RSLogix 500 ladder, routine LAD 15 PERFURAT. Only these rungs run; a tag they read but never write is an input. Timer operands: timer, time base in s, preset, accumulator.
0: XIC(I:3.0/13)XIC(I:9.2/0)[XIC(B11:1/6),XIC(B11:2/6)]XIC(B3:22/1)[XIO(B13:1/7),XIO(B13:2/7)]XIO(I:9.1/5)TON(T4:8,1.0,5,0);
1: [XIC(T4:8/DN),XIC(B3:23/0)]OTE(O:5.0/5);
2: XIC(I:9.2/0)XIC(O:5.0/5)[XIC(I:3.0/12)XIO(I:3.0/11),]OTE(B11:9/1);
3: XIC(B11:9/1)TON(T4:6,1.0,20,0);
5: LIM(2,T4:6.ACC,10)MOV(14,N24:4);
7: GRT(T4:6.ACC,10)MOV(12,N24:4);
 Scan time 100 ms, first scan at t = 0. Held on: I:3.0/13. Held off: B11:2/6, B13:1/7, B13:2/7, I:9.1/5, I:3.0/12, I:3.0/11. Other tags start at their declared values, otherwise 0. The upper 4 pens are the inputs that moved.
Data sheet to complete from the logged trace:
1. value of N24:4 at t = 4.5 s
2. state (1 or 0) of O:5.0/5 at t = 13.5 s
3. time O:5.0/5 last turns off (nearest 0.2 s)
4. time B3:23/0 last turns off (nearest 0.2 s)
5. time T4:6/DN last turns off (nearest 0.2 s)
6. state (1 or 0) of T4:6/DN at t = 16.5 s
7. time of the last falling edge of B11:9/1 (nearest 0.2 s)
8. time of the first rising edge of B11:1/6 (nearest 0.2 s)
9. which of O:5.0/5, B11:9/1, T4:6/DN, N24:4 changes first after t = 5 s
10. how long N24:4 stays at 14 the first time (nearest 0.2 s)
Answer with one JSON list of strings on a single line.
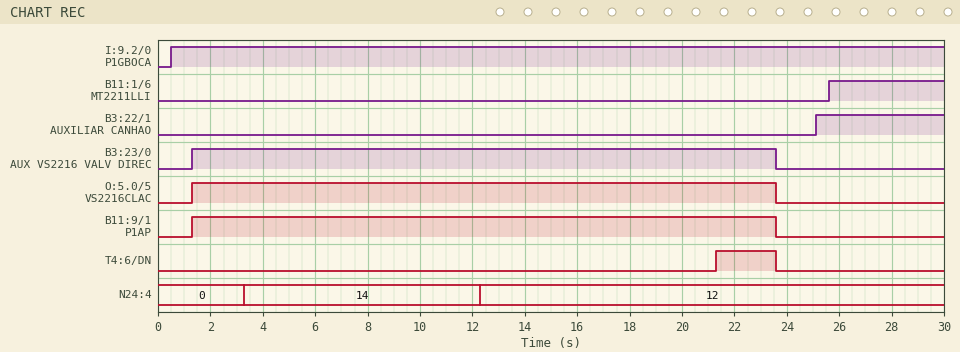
["14", "1", "23.6 s", "23.6 s", "23.6 s", "0", "23.6 s", "25.6 s", "N24:4", "9.0 s"]
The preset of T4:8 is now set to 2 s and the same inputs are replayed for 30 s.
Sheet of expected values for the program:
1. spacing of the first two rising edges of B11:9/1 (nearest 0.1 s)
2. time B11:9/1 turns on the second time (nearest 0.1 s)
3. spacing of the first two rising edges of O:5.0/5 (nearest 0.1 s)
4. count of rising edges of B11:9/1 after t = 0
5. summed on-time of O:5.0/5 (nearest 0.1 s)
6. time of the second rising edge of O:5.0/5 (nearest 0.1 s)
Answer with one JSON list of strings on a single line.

["26.3 s", "27.6 s", "26.3 s", "2", "24.7 s", "27.6 s"]
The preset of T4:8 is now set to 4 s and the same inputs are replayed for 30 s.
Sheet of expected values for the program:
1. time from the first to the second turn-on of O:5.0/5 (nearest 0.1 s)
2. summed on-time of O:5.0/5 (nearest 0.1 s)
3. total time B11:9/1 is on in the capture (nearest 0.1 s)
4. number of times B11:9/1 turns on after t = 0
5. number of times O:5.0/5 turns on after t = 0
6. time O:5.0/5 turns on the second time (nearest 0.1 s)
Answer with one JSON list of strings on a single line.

["28.3 s", "22.7 s", "22.7 s", "2", "2", "29.6 s"]
